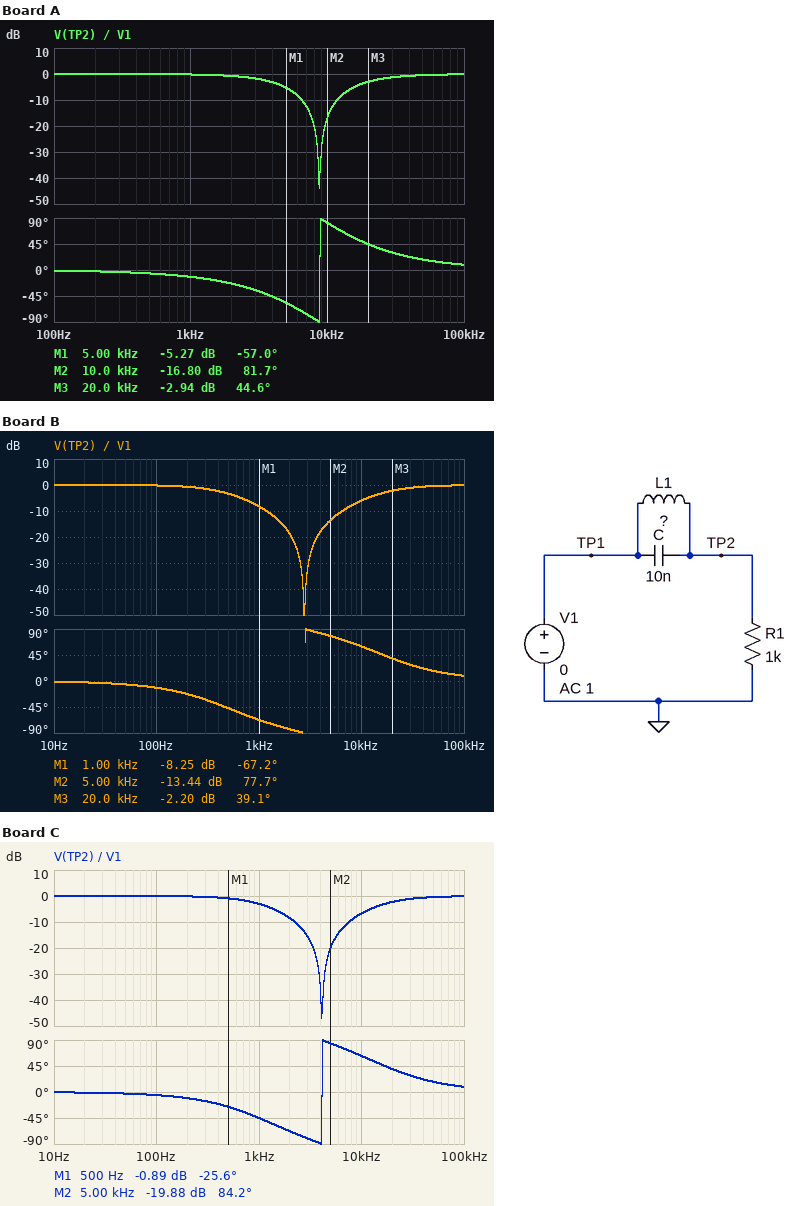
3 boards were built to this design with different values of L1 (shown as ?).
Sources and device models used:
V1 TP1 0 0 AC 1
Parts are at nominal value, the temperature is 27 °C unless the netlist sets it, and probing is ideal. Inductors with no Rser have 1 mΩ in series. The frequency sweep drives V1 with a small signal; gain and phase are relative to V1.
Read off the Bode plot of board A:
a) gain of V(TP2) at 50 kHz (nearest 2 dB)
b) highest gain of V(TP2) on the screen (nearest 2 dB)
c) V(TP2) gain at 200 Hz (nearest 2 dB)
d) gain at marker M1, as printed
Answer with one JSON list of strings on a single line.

["0 dB", "0 dB", "0 dB", "-5.27 dB"]
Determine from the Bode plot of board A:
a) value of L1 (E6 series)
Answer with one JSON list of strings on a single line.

["33 mH"]
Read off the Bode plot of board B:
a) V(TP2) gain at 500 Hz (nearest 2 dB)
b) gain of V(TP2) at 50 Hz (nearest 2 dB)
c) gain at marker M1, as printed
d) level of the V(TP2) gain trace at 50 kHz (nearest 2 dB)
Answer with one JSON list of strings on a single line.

["-4 dB", "0 dB", "-8.25 dB", "0 dB"]
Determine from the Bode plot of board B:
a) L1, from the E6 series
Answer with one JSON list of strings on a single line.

["330 mH"]
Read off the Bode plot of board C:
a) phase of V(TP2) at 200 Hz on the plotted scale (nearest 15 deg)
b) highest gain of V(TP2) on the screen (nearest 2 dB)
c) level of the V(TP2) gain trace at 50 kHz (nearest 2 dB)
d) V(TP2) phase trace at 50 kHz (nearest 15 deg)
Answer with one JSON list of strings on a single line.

["-15 deg", "0 dB", "0 dB", "15 deg"]
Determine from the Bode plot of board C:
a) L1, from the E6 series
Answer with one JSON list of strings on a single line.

["150 mH"]
